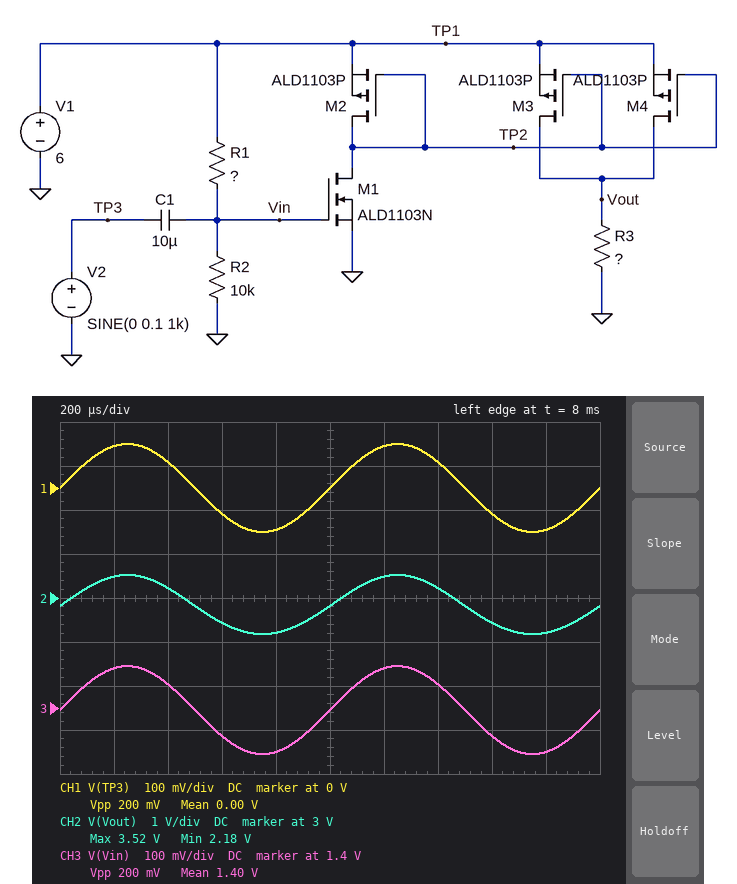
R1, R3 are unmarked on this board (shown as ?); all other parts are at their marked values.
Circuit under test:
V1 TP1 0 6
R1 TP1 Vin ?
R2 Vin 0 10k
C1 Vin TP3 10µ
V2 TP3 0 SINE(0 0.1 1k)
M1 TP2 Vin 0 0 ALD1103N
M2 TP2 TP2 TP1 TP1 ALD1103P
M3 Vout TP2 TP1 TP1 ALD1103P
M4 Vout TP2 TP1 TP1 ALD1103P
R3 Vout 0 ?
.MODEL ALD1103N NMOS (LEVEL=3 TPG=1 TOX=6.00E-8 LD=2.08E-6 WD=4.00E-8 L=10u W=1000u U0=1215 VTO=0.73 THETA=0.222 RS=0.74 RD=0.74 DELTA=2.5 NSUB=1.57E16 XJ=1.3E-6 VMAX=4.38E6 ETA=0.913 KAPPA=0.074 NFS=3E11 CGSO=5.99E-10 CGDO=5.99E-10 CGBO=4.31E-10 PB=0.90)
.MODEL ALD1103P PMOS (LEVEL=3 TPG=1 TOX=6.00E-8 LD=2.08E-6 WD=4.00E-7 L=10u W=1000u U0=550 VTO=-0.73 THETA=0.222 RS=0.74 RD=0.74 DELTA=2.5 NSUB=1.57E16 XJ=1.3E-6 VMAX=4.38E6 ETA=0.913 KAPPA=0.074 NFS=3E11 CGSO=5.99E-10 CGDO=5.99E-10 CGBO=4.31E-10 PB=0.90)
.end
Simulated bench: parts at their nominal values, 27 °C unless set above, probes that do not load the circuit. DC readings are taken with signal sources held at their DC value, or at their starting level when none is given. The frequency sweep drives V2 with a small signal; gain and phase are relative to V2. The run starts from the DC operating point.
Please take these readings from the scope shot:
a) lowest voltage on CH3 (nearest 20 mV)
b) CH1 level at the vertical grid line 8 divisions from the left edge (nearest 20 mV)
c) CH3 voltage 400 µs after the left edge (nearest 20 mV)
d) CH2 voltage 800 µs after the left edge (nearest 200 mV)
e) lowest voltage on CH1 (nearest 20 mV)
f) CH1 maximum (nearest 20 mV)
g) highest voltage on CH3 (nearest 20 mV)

1.30 V
-60 mV
1.46 V
2.2 V
-100 mV
100 mV
1.50 V
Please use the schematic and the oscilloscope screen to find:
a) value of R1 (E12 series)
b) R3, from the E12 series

33 kΩ
680 Ω
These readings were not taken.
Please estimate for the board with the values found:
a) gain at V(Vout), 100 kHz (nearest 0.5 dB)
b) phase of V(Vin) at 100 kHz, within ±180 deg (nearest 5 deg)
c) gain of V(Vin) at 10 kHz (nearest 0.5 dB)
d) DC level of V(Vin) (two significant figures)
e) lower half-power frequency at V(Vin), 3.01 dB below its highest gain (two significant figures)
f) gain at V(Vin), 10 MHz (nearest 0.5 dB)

16.5 dB
0 deg
0 dB
1.4 V
2.1 Hz
0 dB
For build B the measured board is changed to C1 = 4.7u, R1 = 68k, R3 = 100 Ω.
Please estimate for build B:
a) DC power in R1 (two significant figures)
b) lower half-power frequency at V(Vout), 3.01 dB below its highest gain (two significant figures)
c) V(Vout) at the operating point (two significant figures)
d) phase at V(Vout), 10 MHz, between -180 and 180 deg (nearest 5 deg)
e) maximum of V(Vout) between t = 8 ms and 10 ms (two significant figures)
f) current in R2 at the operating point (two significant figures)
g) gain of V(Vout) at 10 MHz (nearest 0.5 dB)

400 µW
3.9 Hz
17 mV
-50 deg
47 mV
77 µA
-15.5 dB
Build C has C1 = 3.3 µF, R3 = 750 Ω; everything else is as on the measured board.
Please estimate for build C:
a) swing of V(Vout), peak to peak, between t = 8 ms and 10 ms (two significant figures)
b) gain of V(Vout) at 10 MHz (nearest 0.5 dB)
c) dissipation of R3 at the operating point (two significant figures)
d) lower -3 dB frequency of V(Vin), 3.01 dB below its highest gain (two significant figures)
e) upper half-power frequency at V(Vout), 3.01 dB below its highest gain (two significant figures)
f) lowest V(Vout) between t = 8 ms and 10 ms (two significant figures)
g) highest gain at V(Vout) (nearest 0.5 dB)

1.5 V
17.0 dB
13 mW
6.3 Hz
30 MHz
2.4 V
17.5 dB
